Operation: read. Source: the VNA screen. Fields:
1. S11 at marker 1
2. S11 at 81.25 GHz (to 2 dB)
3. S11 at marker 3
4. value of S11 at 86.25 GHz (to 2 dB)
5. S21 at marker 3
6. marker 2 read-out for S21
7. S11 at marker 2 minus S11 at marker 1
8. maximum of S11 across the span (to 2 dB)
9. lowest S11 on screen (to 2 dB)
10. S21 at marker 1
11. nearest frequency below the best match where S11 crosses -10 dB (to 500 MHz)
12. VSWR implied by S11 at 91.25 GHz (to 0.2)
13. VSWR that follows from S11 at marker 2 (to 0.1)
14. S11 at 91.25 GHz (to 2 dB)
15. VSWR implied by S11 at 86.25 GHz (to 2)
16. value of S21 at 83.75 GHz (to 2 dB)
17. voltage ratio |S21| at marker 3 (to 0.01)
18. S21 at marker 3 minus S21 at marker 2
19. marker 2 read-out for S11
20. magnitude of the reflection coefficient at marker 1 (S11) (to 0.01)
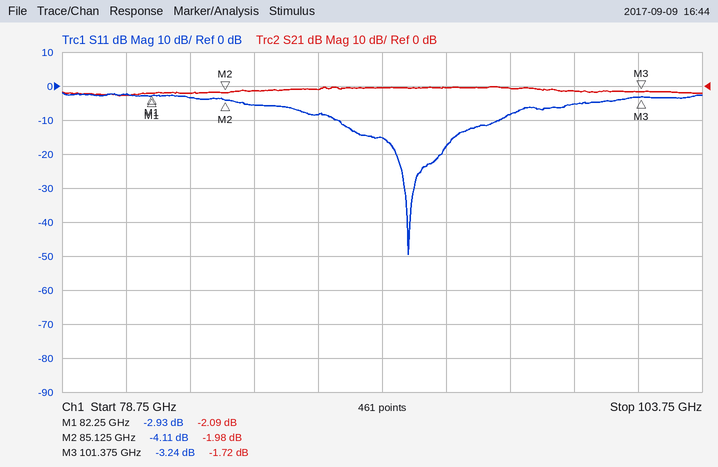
-2.93 dB
-2 dB
-3.24 dB
-6 dB
-1.72 dB
-1.98 dB
-1.18 dB
-2 dB
-50 dB
-2.09 dB
89.5 GHz
1.4
4.3
-16 dB
4
-2 dB
0.82
0.26 dB
-4.11 dB
0.71
